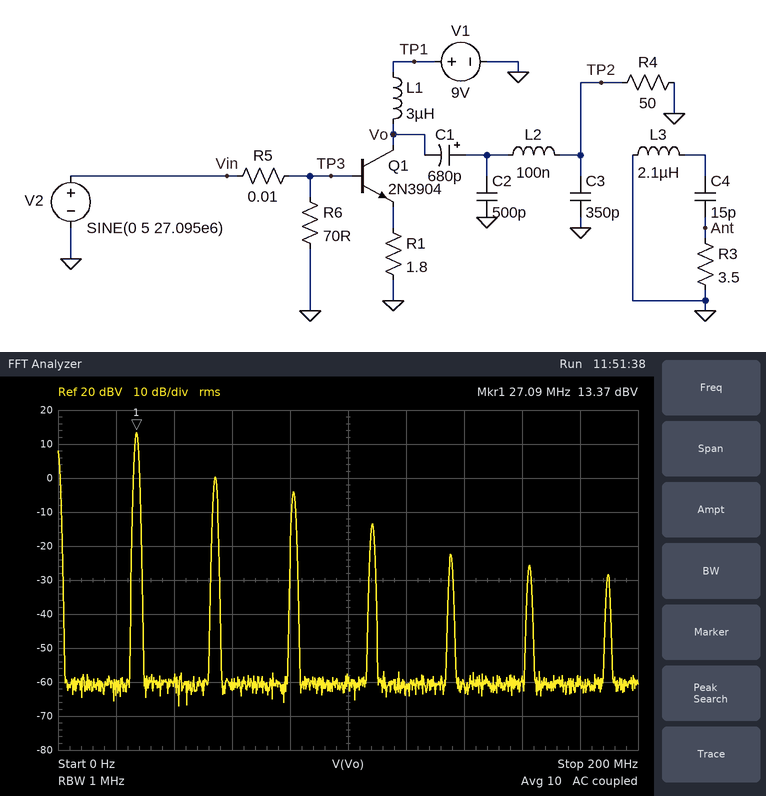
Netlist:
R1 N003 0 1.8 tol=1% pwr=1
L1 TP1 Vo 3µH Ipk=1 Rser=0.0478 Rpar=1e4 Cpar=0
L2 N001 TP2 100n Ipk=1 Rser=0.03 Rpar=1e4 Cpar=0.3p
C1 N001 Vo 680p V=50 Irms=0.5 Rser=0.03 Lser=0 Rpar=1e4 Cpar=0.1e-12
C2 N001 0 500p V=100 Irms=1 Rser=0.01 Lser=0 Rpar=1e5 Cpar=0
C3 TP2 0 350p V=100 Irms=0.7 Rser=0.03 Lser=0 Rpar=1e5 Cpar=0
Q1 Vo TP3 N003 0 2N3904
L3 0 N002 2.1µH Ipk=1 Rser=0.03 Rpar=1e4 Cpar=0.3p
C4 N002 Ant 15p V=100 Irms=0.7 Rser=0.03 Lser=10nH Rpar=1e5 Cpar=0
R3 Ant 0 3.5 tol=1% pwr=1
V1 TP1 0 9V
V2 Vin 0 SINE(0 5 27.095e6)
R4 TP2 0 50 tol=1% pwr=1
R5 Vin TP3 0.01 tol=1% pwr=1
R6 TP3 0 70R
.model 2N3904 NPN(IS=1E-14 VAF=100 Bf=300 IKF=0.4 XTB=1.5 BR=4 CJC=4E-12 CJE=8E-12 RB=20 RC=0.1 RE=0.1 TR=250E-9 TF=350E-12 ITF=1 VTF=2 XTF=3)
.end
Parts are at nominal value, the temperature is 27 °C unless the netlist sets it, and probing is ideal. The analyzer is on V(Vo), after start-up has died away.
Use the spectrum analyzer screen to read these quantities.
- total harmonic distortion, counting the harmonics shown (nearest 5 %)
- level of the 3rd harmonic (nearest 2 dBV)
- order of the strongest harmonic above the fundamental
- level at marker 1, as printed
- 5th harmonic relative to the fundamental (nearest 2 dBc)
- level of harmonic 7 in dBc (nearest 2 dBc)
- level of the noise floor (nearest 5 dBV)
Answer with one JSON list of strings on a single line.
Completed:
["25 %", "-4 dBV", "2", "13.37 dBV", "-36 dBc", "-42 dBc", "-60 dBV"]
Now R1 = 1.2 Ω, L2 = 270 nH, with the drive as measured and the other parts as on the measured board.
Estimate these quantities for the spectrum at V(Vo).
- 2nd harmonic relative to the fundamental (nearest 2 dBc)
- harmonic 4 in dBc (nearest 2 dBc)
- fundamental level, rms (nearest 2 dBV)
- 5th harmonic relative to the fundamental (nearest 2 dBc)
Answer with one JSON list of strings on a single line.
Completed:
["-12 dBc", "-30 dBc", "18 dBV", "-32 dBc"]
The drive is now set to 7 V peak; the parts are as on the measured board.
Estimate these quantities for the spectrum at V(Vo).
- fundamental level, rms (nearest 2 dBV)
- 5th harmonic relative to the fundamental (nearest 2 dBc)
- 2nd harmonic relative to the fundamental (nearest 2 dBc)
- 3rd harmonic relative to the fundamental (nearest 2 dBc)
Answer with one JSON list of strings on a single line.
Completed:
["16 dBV", "-30 dBc", "-18 dBc", "-14 dBc"]
